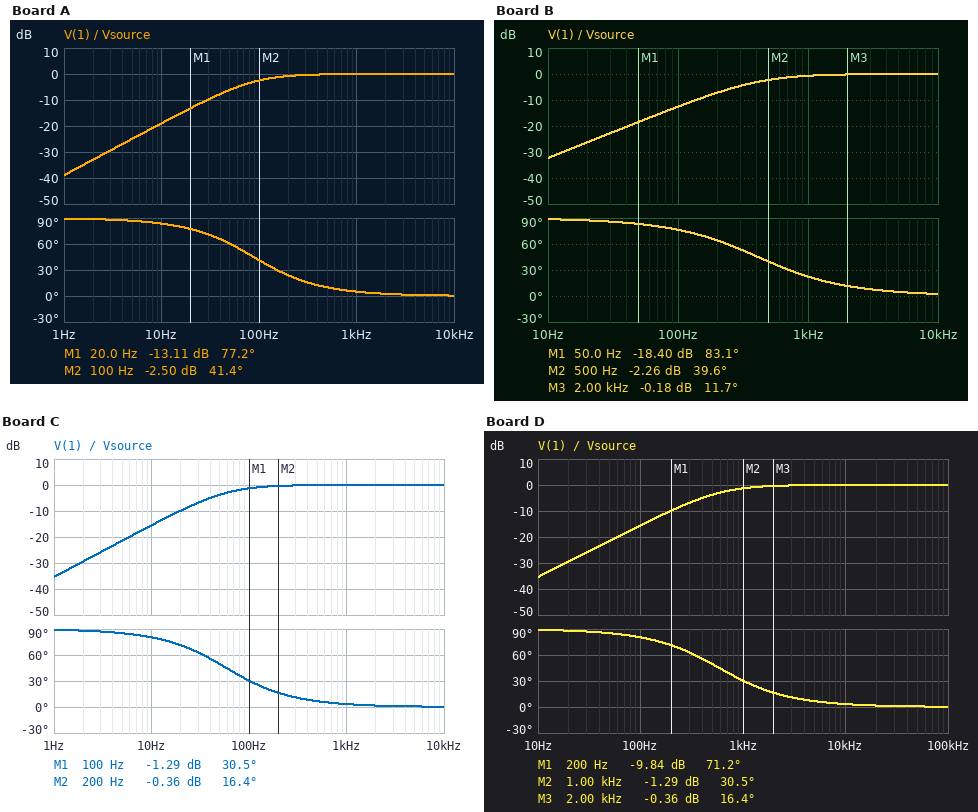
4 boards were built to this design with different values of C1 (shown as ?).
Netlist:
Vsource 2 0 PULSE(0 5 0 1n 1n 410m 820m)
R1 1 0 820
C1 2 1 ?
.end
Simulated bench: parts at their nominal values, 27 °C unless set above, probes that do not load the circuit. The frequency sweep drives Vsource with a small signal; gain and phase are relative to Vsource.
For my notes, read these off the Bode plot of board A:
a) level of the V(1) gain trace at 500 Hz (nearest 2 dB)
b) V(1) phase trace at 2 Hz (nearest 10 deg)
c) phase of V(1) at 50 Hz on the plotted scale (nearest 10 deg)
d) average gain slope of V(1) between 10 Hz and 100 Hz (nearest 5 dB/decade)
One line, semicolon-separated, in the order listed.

0 dB; 90 deg; 60 deg; 15 dB/decade
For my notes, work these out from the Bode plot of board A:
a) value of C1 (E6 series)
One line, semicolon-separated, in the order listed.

2.2 µF
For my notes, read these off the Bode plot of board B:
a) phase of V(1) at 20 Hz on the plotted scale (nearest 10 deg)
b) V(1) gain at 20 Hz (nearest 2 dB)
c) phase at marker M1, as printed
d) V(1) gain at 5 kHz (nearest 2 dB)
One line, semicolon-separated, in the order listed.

90 deg; -26 dB; 83.1 deg; 0 dB
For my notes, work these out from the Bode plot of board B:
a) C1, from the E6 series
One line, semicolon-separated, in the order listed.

470 nF
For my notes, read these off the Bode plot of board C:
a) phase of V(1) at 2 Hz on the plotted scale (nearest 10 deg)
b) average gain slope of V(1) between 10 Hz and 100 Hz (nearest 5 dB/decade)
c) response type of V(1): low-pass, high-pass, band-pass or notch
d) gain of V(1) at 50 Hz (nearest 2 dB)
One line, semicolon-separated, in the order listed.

90 deg; 15 dB/decade; high-pass; -4 dB
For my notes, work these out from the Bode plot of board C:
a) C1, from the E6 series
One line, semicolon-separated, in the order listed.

3.3 µF
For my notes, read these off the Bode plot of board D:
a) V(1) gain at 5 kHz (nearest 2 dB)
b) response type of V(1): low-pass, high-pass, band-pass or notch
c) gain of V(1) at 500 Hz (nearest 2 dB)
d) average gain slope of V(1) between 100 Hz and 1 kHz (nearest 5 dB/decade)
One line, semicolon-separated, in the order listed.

0 dB; high-pass; -4 dB; 15 dB/decade
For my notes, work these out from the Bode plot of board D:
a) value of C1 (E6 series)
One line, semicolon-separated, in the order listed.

330 nF
